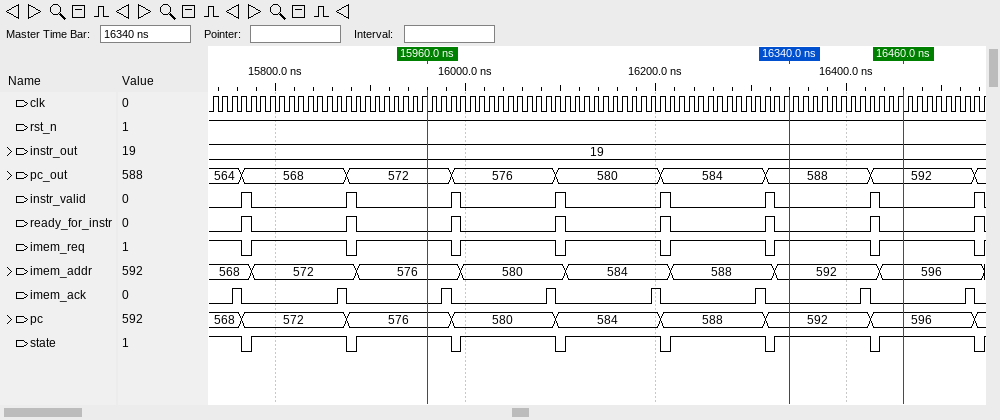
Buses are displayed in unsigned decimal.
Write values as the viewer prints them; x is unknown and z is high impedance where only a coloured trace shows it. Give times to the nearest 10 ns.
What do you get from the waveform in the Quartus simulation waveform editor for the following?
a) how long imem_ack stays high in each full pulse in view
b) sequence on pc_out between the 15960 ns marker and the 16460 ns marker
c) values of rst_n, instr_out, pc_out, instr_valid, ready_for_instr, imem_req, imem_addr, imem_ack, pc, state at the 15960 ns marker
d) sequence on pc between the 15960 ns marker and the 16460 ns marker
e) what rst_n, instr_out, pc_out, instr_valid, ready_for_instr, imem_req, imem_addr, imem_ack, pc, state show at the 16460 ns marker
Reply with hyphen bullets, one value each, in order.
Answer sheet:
- 10 ns, 10 ns, 10 ns, 10 ns, 10 ns, 10 ns, 10 ns, 10 ns
- 572, 576, 580, 584, 588, 592
- rst_n=1, instr_out=19, pc_out=572, instr_valid=0, ready_for_instr=0, imem_req=1, imem_addr=576, imem_ack=0, pc=576, state=1
- 576, 580, 584, 588, 592, 596
- rst_n=1, instr_out=19, pc_out=592, instr_valid=0, ready_for_instr=0, imem_req=1, imem_addr=596, imem_ack=0, pc=596, state=1
